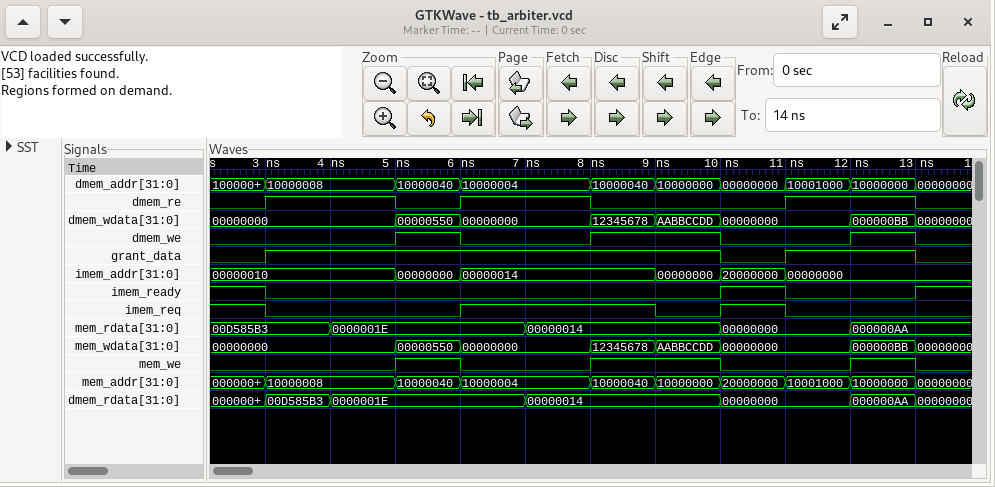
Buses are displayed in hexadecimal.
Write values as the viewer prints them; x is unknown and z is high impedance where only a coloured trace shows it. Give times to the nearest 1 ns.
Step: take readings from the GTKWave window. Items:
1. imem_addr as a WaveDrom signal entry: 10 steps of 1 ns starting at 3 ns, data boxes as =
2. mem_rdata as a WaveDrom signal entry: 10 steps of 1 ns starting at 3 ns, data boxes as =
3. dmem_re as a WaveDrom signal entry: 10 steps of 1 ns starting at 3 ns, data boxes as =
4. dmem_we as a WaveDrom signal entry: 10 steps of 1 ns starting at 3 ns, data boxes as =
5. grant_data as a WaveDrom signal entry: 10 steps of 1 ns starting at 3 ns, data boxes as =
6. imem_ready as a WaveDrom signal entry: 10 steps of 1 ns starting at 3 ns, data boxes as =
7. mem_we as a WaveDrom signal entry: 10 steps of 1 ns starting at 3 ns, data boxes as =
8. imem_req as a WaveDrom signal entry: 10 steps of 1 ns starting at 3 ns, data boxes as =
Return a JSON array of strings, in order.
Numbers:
["{name: 'imem_addr', wave: '=.==..===.', data: '00000010 00000000 00000014 00000000 20000000 00000000'}", "{name: 'mem_rdata', wave: '==..=..=.=', data: '00D585B3 0000001E 00000014 00000000 000000AA'}", "{name: 'dmem_re', wave: '1.01.0..1.'}", "{name: 'dmem_we', wave: '0.10.1.0.1'}", "{name: 'grant_data', wave: '1......01.'}", "{name: 'imem_ready', wave: '0......10.'}", "{name: 'mem_we', wave: '0.10.1.0.1'}", "{name: 'imem_req', wave: '0..1..010.'}"]
